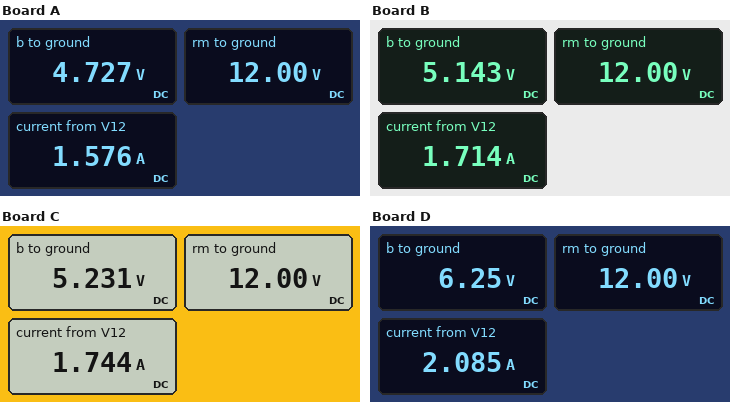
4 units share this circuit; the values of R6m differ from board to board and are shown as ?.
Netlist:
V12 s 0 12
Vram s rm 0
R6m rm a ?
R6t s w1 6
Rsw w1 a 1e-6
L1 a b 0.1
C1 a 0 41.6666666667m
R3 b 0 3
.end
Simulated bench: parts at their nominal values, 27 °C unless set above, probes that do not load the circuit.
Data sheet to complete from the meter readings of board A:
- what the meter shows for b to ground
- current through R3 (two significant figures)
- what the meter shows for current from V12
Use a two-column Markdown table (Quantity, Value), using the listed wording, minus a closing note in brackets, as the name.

| Quantity | Value |
|---|---|
| what the meter shows for b to ground | 4.727 V |
| current through R3 | 1.6 A |
| what the meter shows for current from V12 | 1.576 A |
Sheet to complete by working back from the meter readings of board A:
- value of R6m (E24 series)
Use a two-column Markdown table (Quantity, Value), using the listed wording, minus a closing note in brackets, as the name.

| Quantity | Value |
|---|---|
| value of R6m | 20 Ω |
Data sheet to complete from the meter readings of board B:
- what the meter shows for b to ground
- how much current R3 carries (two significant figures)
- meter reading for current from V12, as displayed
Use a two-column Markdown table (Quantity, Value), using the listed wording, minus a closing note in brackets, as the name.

| Quantity | Value |
|---|---|
| what the meter shows for b to ground | 5.143 V |
| how much current R3 carries | 1.7 A |
| meter reading for current from V12, as displayed | 1.714 A |
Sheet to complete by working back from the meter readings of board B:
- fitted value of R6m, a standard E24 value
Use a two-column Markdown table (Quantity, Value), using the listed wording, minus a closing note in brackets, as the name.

| Quantity | Value |
|---|---|
| fitted value of R6m, a standard E24 value | 12 Ω |
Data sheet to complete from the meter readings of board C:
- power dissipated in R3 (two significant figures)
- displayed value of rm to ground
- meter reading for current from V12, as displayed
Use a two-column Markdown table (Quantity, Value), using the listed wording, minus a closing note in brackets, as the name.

| Quantity | Value |
|---|---|
| power dissipated in R3 | 9.1 W |
| displayed value of rm to ground | 12.00 V |
| meter reading for current from V12, as displayed | 1.744 A |
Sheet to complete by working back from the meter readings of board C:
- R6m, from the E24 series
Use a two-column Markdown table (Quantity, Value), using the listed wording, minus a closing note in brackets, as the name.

| Quantity | Value |
|---|---|
| R6m, from the E24 series | 11 Ω |
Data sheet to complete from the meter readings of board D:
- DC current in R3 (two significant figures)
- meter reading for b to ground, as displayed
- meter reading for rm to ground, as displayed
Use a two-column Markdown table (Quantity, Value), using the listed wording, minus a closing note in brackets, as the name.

| Quantity | Value |
|---|---|
| DC current in R3 | 2.1 A |
| meter reading for b to ground, as displayed | 6.25 V |
| meter reading for rm to ground, as displayed | 12.00 V |
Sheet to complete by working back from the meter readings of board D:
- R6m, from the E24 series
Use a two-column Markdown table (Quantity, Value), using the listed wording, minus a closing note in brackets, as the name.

| Quantity | Value |
|---|---|
| R6m, from the E24 series | 5.1 Ω |
